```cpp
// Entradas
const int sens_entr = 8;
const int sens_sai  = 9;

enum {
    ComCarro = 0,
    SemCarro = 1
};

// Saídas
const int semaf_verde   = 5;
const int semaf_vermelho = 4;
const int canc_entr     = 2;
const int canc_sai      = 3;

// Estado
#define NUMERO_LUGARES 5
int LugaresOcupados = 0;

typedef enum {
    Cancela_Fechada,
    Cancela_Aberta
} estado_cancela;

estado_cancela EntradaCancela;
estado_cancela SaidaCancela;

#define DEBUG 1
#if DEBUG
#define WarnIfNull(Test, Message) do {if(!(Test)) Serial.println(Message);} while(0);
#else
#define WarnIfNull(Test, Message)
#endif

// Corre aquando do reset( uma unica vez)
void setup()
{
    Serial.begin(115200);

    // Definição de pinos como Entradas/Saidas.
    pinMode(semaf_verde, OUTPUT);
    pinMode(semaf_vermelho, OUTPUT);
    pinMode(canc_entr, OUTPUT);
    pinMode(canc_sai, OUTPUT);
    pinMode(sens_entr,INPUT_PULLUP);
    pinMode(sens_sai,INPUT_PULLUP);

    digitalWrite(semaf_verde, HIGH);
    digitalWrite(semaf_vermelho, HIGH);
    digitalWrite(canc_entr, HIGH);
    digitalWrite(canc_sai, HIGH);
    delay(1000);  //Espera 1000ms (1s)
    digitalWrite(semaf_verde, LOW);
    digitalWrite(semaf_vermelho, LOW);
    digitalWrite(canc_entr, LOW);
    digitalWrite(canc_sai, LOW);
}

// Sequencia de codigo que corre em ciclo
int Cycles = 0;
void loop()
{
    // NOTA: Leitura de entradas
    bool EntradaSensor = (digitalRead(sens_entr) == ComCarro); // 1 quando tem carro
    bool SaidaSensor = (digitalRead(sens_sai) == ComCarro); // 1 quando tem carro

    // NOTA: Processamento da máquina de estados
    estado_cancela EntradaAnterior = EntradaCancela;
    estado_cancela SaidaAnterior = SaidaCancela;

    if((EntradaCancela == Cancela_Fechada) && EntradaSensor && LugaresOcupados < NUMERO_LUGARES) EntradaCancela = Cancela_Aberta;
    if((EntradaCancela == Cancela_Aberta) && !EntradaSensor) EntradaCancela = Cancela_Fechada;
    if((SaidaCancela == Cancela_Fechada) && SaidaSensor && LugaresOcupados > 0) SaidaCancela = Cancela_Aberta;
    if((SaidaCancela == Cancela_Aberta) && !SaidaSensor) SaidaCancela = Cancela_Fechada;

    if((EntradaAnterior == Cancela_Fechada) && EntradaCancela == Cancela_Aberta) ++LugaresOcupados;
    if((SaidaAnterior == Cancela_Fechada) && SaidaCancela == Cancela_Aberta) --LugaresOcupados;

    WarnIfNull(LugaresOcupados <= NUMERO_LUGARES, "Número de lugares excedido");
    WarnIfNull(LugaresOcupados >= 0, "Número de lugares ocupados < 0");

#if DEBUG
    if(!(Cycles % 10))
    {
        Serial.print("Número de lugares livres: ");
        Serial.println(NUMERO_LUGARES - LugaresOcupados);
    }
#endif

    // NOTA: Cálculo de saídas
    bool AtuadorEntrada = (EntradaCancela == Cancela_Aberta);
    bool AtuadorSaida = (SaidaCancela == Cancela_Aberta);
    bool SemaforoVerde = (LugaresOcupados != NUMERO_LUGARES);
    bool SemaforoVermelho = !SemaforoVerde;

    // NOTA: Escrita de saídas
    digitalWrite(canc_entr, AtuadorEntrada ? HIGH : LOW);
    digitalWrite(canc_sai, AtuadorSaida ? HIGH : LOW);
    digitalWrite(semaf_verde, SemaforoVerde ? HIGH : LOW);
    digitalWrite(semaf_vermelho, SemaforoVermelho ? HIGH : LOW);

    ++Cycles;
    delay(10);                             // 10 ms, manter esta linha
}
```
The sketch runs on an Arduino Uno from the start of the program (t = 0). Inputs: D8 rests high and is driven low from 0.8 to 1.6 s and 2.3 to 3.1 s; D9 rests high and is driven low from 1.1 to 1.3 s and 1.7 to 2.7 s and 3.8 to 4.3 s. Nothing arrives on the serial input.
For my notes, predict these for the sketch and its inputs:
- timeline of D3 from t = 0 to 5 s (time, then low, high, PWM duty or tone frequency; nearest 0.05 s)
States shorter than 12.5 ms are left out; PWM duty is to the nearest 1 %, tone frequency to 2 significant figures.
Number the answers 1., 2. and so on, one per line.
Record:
1. 0 s high; 1 s low; 1.1 s high; 1.3 s low; 2.3 s high; 2.7 s low
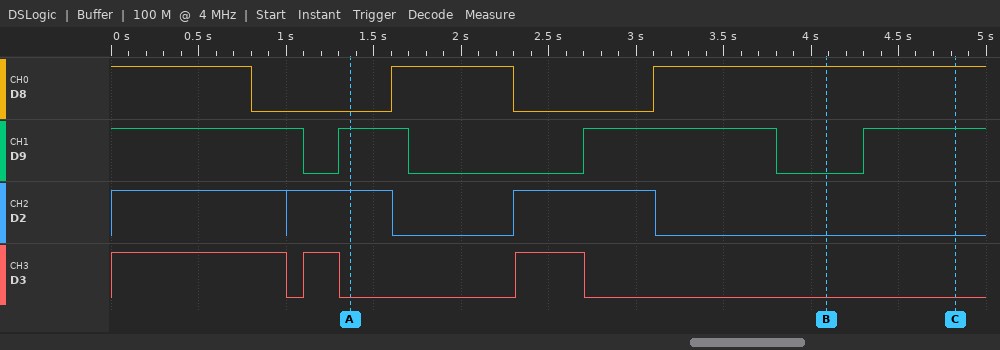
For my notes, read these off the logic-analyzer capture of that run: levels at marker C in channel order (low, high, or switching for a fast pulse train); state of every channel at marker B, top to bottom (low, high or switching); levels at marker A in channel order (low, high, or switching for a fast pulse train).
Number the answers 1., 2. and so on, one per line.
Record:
1. D8 high, D9 high, D2 low, D3 low
2. D8 high, D9 low, D2 low, D3 low
3. D8 low, D9 high, D2 high, D3 low
